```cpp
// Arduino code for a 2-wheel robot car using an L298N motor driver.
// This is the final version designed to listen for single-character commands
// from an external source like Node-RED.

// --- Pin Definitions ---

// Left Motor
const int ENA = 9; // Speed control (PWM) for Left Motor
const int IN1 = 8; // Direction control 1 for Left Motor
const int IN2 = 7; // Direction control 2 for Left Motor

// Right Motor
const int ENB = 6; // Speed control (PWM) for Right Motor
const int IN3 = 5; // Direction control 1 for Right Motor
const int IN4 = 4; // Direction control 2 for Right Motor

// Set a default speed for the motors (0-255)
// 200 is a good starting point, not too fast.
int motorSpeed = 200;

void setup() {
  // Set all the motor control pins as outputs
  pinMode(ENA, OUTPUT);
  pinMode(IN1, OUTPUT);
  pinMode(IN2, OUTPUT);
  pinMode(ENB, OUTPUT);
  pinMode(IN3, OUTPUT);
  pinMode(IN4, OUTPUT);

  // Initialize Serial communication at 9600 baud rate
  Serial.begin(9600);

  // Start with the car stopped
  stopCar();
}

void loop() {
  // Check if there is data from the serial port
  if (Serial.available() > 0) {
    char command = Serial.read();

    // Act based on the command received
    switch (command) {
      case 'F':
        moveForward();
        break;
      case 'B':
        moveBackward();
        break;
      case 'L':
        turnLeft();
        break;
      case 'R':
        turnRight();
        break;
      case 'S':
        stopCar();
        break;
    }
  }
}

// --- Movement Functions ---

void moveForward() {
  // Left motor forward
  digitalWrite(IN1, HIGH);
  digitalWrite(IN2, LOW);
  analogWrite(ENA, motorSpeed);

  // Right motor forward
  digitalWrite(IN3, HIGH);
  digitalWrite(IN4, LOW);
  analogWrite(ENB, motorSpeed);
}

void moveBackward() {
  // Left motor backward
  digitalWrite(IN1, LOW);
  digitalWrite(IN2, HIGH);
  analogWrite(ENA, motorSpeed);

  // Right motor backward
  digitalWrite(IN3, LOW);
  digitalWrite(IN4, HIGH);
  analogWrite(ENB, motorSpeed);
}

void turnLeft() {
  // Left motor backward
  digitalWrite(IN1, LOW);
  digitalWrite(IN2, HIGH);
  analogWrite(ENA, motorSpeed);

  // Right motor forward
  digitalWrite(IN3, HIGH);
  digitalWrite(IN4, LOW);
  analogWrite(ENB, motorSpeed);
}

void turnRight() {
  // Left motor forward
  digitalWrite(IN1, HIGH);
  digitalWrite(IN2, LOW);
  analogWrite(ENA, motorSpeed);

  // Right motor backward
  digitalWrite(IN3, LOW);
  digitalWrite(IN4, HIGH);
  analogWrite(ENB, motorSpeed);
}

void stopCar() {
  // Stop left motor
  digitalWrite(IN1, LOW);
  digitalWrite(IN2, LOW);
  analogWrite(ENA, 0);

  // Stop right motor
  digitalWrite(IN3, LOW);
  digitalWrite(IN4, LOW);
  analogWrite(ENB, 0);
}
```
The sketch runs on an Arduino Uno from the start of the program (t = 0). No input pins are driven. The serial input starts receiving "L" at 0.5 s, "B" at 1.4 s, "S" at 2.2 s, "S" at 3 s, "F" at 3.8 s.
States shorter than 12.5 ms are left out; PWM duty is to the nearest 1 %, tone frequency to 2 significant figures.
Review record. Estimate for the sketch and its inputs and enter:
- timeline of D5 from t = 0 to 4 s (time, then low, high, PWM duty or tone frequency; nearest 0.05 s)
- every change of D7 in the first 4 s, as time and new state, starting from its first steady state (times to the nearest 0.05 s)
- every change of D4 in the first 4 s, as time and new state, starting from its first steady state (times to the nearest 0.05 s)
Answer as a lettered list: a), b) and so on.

a) 0 s low; 0.5 s high; 1.4 s low; 3.8 s high
b) 0 s low; 0.5 s high; 2.2 s low
c) 0 s low; 1.4 s high; 2.2 s low
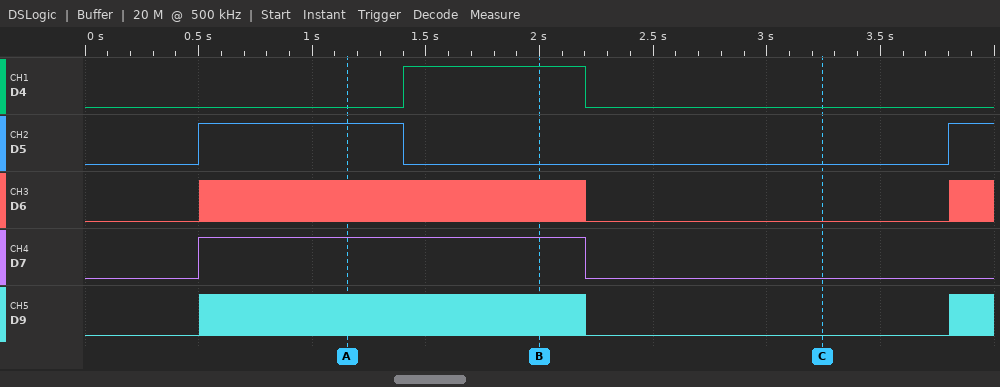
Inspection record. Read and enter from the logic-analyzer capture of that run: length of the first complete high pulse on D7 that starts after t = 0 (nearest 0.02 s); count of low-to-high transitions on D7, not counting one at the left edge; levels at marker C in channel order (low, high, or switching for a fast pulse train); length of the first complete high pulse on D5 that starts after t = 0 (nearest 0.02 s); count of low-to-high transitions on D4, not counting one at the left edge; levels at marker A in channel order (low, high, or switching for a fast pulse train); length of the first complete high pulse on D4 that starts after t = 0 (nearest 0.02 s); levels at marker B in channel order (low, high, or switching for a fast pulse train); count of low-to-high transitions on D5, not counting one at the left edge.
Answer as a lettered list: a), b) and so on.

a) 1.70 s
b) 1
c) D4 low, D5 low, D6 low, D7 low, D9 low
d) 0.90 s
e) 1
f) D4 low, D5 high, D6 switching, D7 high, D9 switching
g) 0.80 s
h) D4 high, D5 low, D6 switching, D7 high, D9 switching
i) 2
